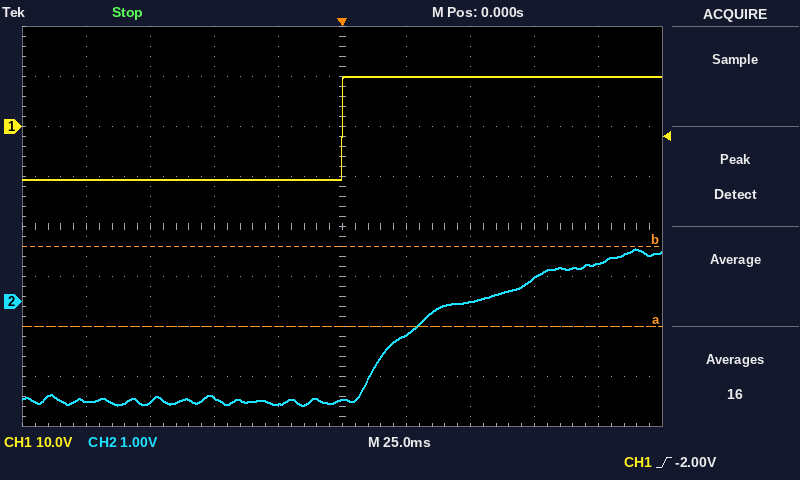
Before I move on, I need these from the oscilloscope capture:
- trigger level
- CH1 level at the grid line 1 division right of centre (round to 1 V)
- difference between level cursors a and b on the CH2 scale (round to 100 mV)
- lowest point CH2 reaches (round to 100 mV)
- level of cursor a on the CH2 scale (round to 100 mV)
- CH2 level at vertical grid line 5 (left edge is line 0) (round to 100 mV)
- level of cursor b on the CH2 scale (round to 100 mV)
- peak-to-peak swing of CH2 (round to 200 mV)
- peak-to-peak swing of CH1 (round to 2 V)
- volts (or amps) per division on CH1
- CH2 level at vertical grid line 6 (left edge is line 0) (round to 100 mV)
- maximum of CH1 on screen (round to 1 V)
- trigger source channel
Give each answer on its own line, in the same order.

-2.00 V
10 V
1.6 V
-2.1 V
-500 mV
-2.0 V
1.1 V
3.2 V
20 V
10 V
-700 mV
10 V
CH1
